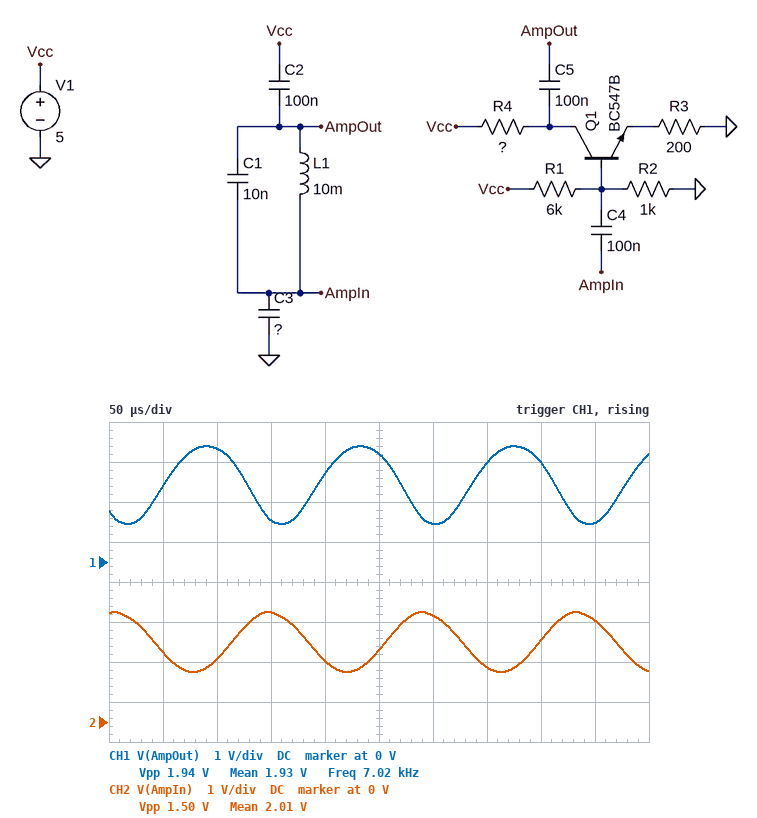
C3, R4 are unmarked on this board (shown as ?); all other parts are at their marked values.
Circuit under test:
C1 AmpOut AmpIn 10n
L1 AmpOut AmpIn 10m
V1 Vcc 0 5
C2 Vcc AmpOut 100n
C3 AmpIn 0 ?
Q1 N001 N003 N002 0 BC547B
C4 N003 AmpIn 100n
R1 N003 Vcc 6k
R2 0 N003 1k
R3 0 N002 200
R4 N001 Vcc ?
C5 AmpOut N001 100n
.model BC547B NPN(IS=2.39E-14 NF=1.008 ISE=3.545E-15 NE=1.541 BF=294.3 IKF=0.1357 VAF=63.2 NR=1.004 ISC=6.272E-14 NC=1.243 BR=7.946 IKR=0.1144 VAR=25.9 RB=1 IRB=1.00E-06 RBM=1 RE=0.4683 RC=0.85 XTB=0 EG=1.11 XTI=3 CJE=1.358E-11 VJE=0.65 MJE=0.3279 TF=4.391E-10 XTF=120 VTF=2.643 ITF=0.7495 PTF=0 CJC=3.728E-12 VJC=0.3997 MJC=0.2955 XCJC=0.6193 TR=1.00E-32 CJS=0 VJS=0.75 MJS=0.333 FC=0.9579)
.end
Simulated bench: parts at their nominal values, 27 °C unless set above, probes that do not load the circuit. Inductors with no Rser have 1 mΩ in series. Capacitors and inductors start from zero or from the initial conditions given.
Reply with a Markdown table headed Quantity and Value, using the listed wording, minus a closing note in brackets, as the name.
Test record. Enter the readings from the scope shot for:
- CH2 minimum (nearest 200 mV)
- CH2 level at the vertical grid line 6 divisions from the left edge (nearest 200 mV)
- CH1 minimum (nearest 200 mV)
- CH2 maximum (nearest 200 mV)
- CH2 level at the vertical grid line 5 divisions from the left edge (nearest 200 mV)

| Quantity | Value |
|---|---|
| CH2 minimum | 1.2 V |
| CH2 level at the vertical grid line 6 divisions from the left edge | 2.6 V |
| CH1 minimum | 1.0 V |
| CH2 maximum | 2.8 V |
| CH2 level at the vertical grid line 5 divisions from the left edge | 1.8 V |
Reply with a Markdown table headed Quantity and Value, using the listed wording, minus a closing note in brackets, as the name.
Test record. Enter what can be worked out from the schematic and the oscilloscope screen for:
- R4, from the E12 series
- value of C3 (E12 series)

| Quantity | Value |
|---|---|
| R4, from the E12 series | 2.7 kΩ |
| value of C3 | 82 nF |
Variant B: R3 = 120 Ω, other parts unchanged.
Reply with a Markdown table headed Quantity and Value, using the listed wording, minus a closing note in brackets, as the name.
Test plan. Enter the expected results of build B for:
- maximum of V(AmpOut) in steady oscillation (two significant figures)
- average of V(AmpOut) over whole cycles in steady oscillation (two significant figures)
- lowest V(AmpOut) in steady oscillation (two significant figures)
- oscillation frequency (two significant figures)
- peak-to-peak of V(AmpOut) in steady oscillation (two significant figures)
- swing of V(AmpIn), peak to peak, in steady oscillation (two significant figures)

| Quantity | Value |
|---|---|
| maximum of V(AmpOut) in steady oscillation | 2.8 V |
| average of V(AmpOut) over whole cycles in steady oscillation | 1.9 V |
| lowest V(AmpOut) in steady oscillation | 930 mV |
| oscillation frequency | 7.2 kHz |
| peak-to-peak of V(AmpOut) in steady oscillation | 1.8 V |
| swing of V(AmpIn), peak to peak, in steady oscillation | 1.2 V |
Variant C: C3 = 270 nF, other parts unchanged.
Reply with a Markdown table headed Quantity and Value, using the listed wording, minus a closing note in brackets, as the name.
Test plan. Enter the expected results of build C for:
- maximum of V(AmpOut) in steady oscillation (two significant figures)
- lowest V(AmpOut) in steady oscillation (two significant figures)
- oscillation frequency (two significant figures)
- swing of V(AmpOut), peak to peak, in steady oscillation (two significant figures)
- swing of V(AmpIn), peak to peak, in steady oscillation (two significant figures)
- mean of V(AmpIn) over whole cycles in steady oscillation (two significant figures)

| Quantity | Value |
|---|---|
| maximum of V(AmpOut) in steady oscillation | 3.4 V |
| lowest V(AmpOut) in steady oscillation | -550 mV |
| oscillation frequency | 5.7 kHz |
| swing of V(AmpOut), peak to peak, in steady oscillation | 3.9 V |
| swing of V(AmpIn), peak to peak, in steady oscillation | 1.2 V |
| mean of V(AmpIn) over whole cycles in steady oscillation | 1.5 V |
